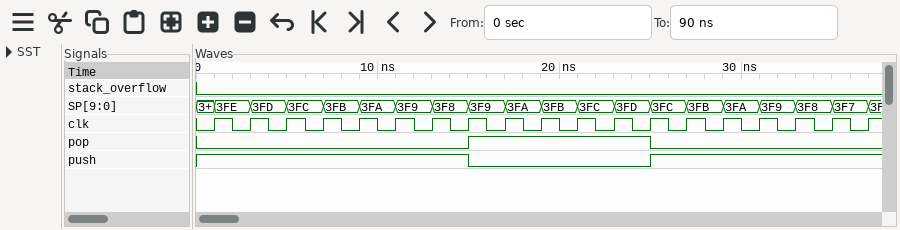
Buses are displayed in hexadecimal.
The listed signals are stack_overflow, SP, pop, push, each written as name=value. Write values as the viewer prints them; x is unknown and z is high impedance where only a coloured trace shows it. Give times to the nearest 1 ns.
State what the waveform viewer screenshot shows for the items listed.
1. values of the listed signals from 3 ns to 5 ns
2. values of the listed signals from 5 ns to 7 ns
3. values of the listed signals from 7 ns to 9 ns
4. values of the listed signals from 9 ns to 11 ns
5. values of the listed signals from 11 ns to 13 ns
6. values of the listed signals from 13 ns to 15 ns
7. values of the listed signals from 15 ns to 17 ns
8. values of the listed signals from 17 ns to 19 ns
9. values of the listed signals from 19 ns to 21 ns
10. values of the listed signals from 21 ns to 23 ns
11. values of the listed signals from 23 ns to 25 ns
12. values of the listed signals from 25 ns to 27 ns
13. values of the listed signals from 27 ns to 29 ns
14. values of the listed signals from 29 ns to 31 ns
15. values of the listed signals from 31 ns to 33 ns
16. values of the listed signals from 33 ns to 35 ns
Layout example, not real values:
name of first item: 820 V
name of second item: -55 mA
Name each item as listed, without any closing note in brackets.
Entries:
values of the listed signals from 3 ns to 5 ns: stack_overflow=0, SP=3FD, pop=0, push=1
values of the listed signals from 5 ns to 7 ns: stack_overflow=0, SP=3FC, pop=0, push=1
values of the listed signals from 7 ns to 9 ns: stack_overflow=0, SP=3FB, pop=0, push=1
values of the listed signals from 9 ns to 11 ns: stack_overflow=0, SP=3FA, pop=0, push=1
values of the listed signals from 11 ns to 13 ns: stack_overflow=0, SP=3F9, pop=0, push=1
values of the listed signals from 13 ns to 15 ns: stack_overflow=0, SP=3F8, pop=0, push=1
values of the listed signals from 15 ns to 17 ns: stack_overflow=0, SP=3F9, pop=1, push=0
values of the listed signals from 17 ns to 19 ns: stack_overflow=0, SP=3FA, pop=1, push=0
values of the listed signals from 19 ns to 21 ns: stack_overflow=0, SP=3FB, pop=1, push=0
values of the listed signals from 21 ns to 23 ns: stack_overflow=0, SP=3FC, pop=1, push=0
values of the listed signals from 23 ns to 25 ns: stack_overflow=0, SP=3FD, pop=1, push=0
values of the listed signals from 25 ns to 27 ns: stack_overflow=0, SP=3FC, pop=0, push=1
values of the listed signals from 27 ns to 29 ns: stack_overflow=0, SP=3FB, pop=0, push=1
values of the listed signals from 29 ns to 31 ns: stack_overflow=0, SP=3FA, pop=0, push=1
values of the listed signals from 31 ns to 33 ns: stack_overflow=0, SP=3F9, pop=0, push=1
values of the listed signals from 33 ns to 35 ns: stack_overflow=0, SP=3F8, pop=0, push=1
